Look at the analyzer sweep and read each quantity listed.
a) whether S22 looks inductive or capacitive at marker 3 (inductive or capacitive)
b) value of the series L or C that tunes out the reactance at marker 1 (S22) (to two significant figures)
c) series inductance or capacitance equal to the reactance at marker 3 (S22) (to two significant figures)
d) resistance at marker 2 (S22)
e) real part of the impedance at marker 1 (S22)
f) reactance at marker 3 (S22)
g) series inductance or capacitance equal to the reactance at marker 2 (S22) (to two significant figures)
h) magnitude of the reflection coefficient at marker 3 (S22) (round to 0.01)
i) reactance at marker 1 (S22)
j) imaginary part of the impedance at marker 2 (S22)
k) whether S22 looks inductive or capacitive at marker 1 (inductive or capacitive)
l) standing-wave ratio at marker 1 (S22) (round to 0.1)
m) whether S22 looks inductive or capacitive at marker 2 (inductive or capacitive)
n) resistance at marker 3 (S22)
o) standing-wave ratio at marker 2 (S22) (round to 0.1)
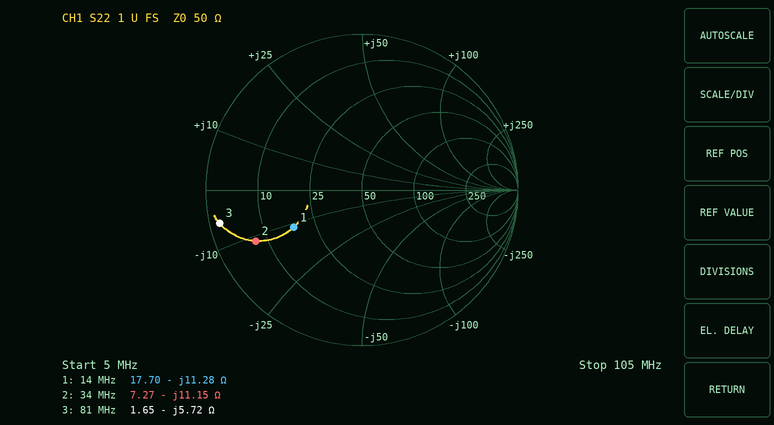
capacitive
130 nH
340 pF
7.27 Ω
17.70 Ω
-5.72 Ω
420 pF
0.94
-11.28 Ω
-11.15 Ω
capacitive
3.0
capacitive
1.65 Ω
7.2
